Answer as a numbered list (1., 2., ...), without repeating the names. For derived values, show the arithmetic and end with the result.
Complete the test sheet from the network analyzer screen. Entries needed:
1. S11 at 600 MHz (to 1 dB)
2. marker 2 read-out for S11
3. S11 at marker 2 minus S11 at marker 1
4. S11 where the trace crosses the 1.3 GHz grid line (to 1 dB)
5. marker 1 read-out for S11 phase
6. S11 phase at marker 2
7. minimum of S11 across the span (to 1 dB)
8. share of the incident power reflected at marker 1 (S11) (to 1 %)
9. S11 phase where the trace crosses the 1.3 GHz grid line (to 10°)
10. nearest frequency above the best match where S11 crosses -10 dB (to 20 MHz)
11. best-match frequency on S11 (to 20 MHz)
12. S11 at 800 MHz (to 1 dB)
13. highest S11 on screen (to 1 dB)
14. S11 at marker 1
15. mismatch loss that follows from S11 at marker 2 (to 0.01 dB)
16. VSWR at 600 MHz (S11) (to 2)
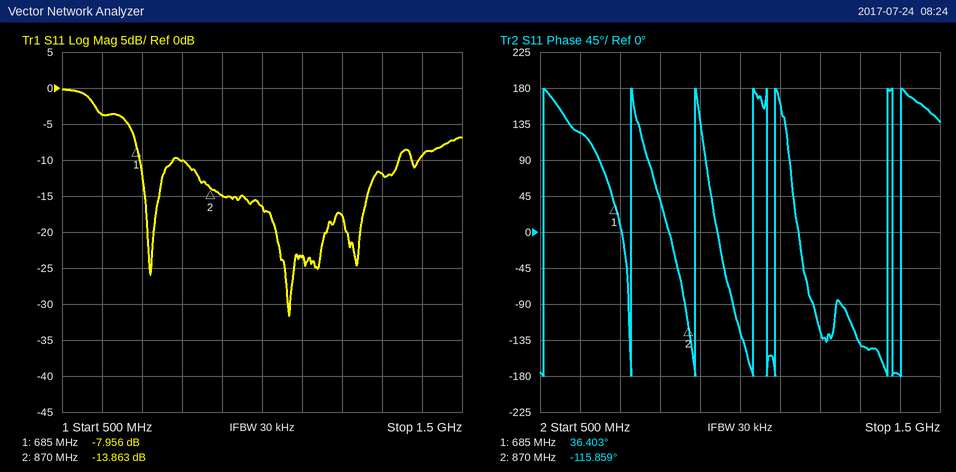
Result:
1. -4 dB
2. -13.863 dB
3. -13.863 − (-7.956) = -5.907 dB
4. -12 dB
5. 36.403°
6. -115.859°
7. -32 dB
8. 10^(-7.956/10) ≈ 16 %
9. -140°
10. 1.34 GHz
11. 1.06 GHz
12. -10 dB
13. 0 dB
14. -7.956 dB
15. −10 log10(1 − 10^(-13.863/10)) ≈ 0.18 dB
16. |Γ| = 10^(-4/20) = 0.6310; VSWR = (1 + 0.6310)/(1 − 0.6310) ≈ 4
